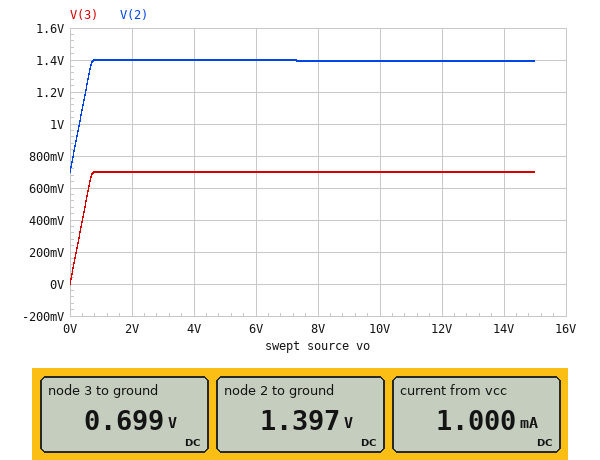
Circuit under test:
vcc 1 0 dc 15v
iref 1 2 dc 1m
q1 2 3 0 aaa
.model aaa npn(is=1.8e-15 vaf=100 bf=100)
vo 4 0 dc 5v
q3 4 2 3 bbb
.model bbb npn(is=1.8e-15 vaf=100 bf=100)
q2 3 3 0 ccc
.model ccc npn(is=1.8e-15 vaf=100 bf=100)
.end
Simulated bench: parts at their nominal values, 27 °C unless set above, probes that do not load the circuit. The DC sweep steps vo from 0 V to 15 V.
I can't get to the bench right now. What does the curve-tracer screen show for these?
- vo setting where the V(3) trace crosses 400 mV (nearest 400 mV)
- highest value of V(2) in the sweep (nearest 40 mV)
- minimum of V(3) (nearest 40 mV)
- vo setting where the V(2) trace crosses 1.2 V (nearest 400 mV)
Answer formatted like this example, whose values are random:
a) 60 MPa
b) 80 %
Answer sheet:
a) 400 mV
b) 1.40 V
c) 0 V
d) 400 mV
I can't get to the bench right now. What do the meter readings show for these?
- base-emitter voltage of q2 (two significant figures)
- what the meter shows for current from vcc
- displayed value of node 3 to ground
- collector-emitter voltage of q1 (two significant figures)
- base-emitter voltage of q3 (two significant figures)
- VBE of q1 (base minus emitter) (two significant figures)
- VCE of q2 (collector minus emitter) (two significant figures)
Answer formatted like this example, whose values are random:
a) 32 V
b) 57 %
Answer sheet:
a) 700 mV
b) 1.000 mA
c) 0.699 V
d) 1.4 V
e) 700 mV
f) 700 mV
g) 700 mV
